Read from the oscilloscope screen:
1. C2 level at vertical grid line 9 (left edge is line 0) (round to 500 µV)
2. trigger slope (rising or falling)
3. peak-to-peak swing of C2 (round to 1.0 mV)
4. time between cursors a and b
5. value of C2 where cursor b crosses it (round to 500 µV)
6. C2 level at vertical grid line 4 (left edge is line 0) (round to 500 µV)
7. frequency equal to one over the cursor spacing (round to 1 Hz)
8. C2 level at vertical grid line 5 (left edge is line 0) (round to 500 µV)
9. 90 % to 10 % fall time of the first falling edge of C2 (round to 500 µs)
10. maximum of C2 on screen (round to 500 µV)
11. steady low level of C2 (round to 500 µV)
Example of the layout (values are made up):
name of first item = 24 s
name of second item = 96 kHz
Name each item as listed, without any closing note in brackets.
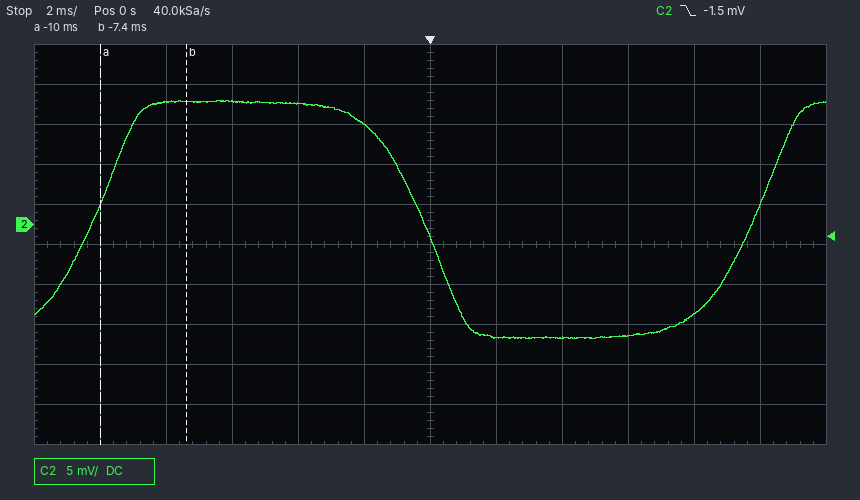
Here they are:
C2 level at vertical grid line 9 (left edge is line 0) = -14.0 mV
trigger slope = falling
peak-to-peak swing of C2 = 30.0 mV
time between cursors a and b = 2.6 ms
value of C2 where cursor b crosses it = 15.5 mV
C2 level at vertical grid line 4 (left edge is line 0) = 15.0 mV
frequency equal to one over the cursor spacing = 385 Hz
C2 level at vertical grid line 5 (left edge is line 0) = 12.5 mV
90 % to 10 % fall time of the first falling edge of C2 = 3.0 ms
maximum of C2 on screen = 15.5 mV
steady low level of C2 = -14.0 mV
